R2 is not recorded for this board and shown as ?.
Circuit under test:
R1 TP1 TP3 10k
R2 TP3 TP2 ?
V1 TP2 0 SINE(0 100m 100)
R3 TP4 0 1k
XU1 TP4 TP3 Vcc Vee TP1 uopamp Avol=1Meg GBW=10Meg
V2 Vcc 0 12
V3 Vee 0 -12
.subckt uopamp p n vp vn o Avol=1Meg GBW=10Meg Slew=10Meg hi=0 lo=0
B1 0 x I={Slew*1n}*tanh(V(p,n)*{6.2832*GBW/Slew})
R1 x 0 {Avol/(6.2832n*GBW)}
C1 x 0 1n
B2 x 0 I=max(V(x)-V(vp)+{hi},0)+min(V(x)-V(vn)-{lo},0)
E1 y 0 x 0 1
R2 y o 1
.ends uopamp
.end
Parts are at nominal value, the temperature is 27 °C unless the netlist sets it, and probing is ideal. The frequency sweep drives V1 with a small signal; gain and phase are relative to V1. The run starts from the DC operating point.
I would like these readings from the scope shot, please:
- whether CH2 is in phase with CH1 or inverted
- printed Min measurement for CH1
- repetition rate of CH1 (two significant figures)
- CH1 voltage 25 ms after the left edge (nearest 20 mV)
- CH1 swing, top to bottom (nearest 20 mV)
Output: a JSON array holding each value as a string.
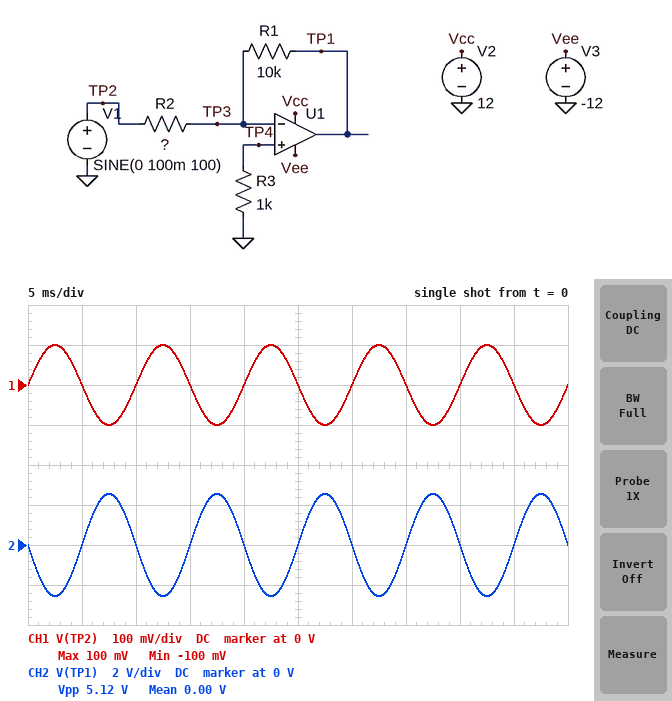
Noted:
["inverted", "-100 mV", "100 Hz", "0 V", "200 mV"]
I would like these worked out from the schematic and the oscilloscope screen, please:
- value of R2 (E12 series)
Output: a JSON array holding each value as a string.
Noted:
["390 Ω"]
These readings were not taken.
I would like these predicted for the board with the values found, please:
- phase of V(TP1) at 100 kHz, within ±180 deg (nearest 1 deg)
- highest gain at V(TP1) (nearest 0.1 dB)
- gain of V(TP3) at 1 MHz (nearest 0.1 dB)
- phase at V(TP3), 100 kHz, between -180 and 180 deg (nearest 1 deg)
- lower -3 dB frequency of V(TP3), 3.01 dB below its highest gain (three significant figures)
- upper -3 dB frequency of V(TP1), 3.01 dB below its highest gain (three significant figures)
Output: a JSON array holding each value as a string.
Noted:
["165 deg", "28.2 dB", "-0.9 dB", "75 deg", "375 kHz", "375 kHz"]
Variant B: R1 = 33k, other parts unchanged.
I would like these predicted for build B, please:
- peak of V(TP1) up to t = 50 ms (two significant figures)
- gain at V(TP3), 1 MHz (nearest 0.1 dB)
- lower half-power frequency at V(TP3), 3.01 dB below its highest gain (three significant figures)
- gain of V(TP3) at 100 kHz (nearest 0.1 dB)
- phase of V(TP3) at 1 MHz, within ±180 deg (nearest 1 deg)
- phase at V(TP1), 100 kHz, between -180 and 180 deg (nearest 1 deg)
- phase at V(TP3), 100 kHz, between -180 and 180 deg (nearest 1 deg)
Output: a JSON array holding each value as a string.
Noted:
["8.5 V", "-0.2 dB", "117 kHz", "-3.8 dB", "7 deg", "139 deg", "49 deg"]
